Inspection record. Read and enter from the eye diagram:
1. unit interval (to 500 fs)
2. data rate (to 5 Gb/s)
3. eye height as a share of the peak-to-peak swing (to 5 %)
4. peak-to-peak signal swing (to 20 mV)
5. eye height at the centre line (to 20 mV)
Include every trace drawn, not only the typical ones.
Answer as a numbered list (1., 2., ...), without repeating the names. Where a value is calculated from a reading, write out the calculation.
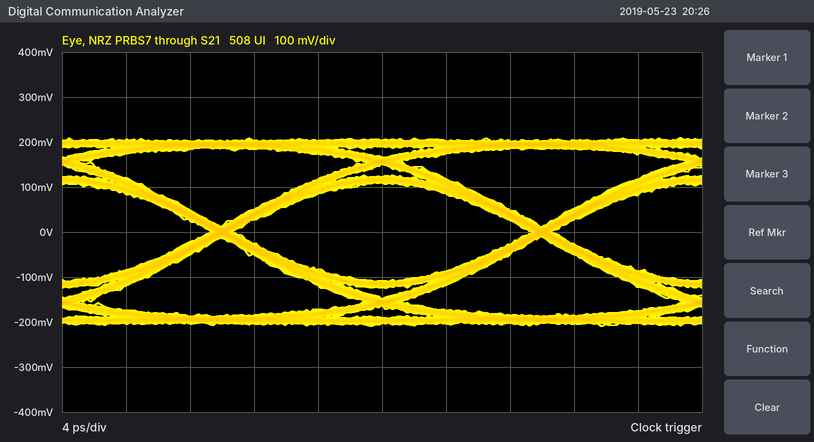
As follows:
1. 20.0 ps
2. 50 Gb/s
3. 220 mV / 420 mV ≈ 52.4 %, so 50 % to the nearest 5 %
4. 420 mV
5. 220 mV
